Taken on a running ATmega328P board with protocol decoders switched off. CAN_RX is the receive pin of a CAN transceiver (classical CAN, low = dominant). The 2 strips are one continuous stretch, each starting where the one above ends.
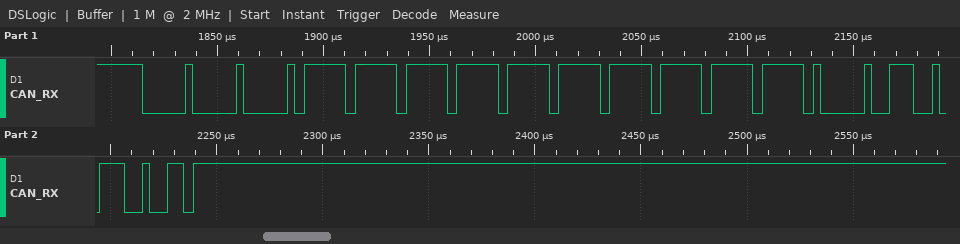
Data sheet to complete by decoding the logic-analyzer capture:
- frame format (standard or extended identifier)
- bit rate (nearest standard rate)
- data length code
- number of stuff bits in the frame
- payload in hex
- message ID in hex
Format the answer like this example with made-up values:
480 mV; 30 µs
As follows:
standard; 250 kbit/s; 7; 14; FF FF FF FF FF FF 01; 0x000
